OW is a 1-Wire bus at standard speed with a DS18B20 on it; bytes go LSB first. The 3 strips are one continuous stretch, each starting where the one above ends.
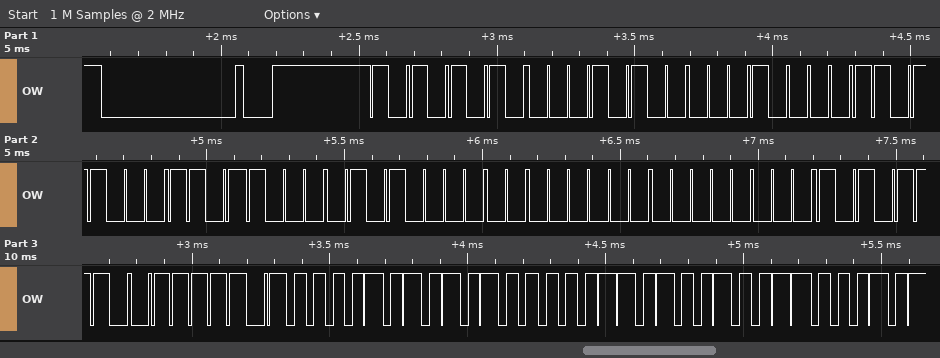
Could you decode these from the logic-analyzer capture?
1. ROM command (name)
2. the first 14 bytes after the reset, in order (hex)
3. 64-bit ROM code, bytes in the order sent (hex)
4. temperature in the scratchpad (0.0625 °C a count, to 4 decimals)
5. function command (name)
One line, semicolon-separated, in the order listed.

Match ROM; 55 28 08 1B 1B 0A 00 00 75 BE 50 05 4B 46; 28 08 1B 1B 0A 00 00 75; 85.0000 °C; Read Scratchpad
